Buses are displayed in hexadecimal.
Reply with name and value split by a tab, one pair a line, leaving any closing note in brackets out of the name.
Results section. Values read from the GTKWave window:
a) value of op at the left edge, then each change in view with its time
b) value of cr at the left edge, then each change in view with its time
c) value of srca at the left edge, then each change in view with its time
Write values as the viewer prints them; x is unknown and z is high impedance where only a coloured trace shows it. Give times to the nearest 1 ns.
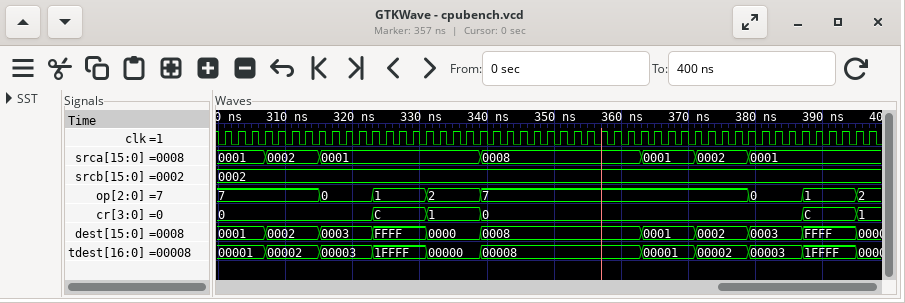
value of op at the left edge, then each change in view with its time	7, 0 at 315 ns, 1 at 323 ns, 2 at 331 ns, 7 at 339 ns, 0 at 379 ns, 1 at 387 ns, 2 at 395 ns
value of cr at the left edge, then each change in view with its time	0, C at 323 ns, 1 at 331 ns, 0 at 339 ns, C at 387 ns, 1 at 395 ns
value of srca at the left edge, then each change in view with its time	0001, 0002 at 307 ns, 0001 at 315 ns, 0008 at 339 ns, 0001 at 363 ns, 0002 at 371 ns, 0001 at 379 ns
